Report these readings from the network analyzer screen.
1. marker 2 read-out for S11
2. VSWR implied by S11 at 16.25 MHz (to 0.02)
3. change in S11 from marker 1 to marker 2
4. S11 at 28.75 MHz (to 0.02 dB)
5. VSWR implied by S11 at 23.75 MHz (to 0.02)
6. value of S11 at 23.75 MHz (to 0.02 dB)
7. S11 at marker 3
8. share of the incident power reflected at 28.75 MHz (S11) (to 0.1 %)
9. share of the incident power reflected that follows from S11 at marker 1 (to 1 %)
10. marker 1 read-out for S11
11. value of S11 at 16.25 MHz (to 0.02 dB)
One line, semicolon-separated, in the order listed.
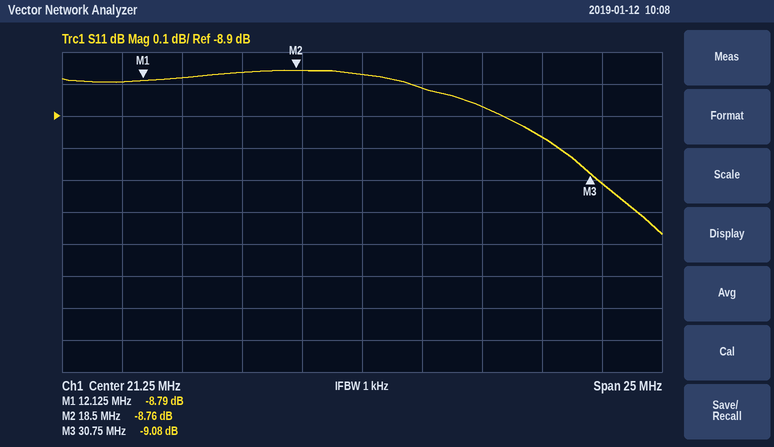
-8.76 dB; 2.14; 0.03 dB; -8.96 dB; 2.14; -8.82 dB; -9.08 dB; 12.7 %; 13 %; -8.79 dB; -8.76 dB
